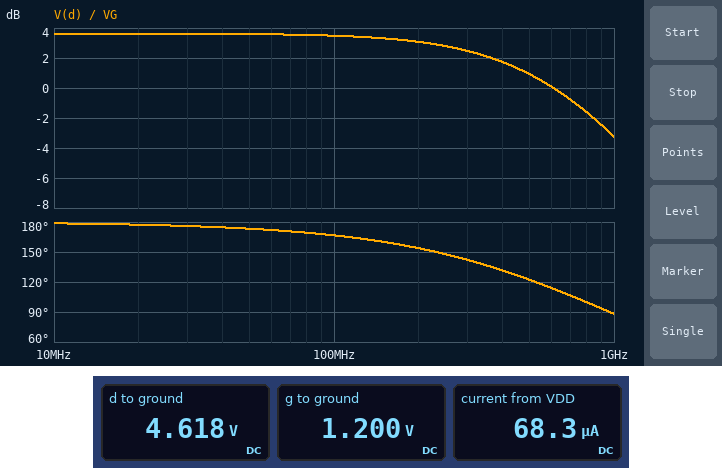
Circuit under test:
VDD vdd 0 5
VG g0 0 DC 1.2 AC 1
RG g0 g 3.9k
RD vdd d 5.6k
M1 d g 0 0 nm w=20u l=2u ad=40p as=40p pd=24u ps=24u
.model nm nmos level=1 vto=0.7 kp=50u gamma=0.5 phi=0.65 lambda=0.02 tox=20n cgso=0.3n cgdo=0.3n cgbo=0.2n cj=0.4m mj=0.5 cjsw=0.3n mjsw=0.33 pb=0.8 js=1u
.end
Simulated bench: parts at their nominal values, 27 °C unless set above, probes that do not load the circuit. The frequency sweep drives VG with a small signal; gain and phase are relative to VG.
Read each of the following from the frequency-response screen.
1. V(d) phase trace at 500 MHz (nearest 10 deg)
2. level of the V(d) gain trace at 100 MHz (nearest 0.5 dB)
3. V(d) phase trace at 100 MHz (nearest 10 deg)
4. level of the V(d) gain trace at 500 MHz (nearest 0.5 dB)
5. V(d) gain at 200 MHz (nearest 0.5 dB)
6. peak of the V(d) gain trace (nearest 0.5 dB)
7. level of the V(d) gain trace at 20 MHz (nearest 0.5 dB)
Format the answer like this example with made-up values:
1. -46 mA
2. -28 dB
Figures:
1. 120 deg
2. 3.5 dB
3. 170 deg
4. 1.0 dB
5. 3.0 dB
6. 3.5 dB
7. 3.5 dB
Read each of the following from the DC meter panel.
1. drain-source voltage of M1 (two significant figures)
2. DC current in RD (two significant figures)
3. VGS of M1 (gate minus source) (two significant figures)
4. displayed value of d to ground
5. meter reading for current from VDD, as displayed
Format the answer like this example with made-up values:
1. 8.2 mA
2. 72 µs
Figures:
1. 4.6 V
2. 68 µA
3. 1.2 V
4. 4.618 V
5. 68.3 µA
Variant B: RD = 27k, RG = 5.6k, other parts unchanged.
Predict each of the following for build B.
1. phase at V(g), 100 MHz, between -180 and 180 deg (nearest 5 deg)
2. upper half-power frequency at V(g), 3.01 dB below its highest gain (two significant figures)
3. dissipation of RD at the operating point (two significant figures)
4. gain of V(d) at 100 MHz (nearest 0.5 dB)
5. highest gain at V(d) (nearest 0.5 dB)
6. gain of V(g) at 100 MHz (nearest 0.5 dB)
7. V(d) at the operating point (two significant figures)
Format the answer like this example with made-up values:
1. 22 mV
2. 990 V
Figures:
1. -20 deg
2. 260 MHz
3. 120 µW
4. 15.5 dB
5. 17.0 dB
6. -1.0 dB
7. 3.2 V
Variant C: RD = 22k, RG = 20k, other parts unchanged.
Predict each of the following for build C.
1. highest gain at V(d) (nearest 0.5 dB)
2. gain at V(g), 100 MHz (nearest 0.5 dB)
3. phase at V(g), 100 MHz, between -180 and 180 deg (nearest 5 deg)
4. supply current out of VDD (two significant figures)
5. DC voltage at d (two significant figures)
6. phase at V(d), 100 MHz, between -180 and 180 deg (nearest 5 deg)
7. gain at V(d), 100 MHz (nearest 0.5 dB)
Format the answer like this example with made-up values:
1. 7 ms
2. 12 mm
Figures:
1. 15.0 dB
2. -4.0 dB
3. -45 deg
4. 67 µA
5. 3.5 V
6. 120 deg
7. 11.0 dB
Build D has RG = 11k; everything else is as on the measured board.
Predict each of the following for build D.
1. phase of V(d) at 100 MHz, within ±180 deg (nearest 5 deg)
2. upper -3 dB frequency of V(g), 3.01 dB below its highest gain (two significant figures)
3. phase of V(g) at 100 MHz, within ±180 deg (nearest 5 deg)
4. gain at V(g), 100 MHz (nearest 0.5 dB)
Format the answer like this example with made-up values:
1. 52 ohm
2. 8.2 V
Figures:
1. 150 deg
2. 210 MHz
3. -25 deg
4. -1.0 dB
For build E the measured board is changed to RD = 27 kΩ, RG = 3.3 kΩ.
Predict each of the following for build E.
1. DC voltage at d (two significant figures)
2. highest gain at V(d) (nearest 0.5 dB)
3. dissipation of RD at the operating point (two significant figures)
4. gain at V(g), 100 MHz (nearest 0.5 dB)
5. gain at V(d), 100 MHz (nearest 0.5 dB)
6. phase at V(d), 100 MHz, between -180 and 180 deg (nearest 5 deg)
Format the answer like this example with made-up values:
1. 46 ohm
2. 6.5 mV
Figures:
1. 3.2 V
2. 17.0 dB
3. 120 µW
4. -0.5 dB
5. 16.0 dB
6. 150 deg
